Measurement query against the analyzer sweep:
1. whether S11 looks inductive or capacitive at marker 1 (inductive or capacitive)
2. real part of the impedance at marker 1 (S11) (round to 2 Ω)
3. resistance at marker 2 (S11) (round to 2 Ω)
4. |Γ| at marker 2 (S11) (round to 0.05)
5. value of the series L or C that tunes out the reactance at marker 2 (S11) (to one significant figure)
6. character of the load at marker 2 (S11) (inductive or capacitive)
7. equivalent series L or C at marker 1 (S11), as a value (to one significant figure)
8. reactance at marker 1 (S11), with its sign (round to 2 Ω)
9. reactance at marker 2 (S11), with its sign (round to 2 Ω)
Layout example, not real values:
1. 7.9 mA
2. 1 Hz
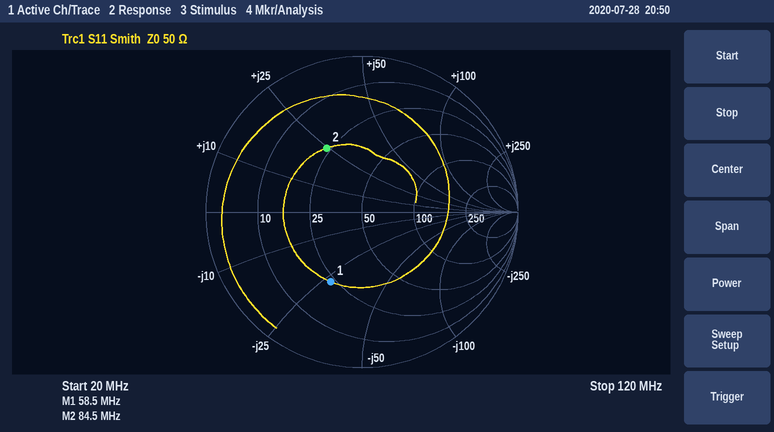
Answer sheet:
1. capacitive
2. 24 Ω
3. 24 Ω
4. 0.45
5. 80 pF
6. inductive
7. 100 pF
8. -28 Ω
9. +24 Ω
